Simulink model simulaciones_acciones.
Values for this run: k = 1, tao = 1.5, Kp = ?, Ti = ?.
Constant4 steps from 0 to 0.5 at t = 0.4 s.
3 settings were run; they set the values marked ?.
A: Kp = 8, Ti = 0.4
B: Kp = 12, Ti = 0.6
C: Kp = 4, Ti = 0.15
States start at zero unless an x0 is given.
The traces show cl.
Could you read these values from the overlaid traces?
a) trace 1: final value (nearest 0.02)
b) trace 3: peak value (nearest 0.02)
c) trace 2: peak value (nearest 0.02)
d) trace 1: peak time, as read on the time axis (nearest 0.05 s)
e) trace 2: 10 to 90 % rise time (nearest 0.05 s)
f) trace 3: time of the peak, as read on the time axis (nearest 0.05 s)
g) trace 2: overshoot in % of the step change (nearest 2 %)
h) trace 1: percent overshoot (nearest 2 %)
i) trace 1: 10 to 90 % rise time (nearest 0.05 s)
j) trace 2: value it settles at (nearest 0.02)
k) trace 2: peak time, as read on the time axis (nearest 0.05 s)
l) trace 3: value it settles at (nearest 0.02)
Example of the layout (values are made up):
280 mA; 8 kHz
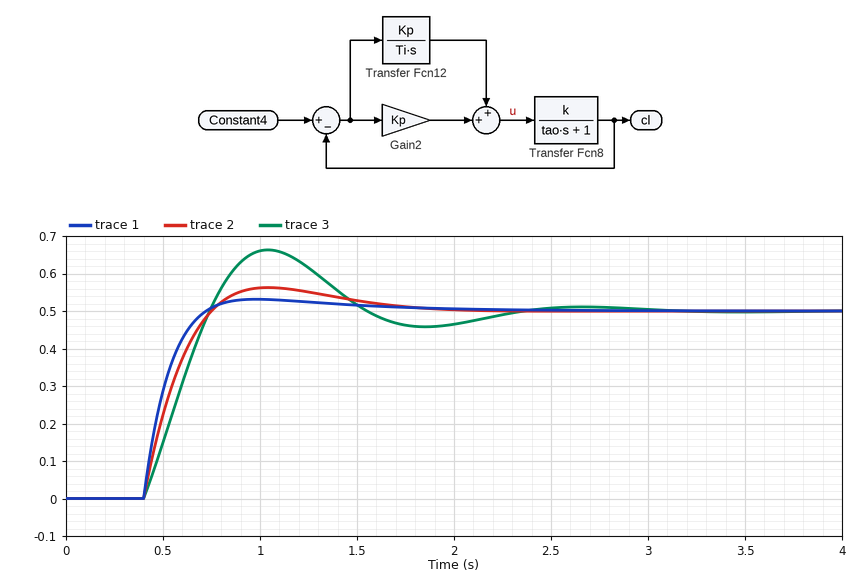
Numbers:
0.50; 0.66; 0.56; 1.00 s; 0.25 s; 1.05 s; 12 %; 6 %; 0.20 s; 0.50; 1.05 s; 0.50
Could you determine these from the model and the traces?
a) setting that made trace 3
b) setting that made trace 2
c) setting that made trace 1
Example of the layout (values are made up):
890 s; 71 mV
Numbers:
C; A; B
